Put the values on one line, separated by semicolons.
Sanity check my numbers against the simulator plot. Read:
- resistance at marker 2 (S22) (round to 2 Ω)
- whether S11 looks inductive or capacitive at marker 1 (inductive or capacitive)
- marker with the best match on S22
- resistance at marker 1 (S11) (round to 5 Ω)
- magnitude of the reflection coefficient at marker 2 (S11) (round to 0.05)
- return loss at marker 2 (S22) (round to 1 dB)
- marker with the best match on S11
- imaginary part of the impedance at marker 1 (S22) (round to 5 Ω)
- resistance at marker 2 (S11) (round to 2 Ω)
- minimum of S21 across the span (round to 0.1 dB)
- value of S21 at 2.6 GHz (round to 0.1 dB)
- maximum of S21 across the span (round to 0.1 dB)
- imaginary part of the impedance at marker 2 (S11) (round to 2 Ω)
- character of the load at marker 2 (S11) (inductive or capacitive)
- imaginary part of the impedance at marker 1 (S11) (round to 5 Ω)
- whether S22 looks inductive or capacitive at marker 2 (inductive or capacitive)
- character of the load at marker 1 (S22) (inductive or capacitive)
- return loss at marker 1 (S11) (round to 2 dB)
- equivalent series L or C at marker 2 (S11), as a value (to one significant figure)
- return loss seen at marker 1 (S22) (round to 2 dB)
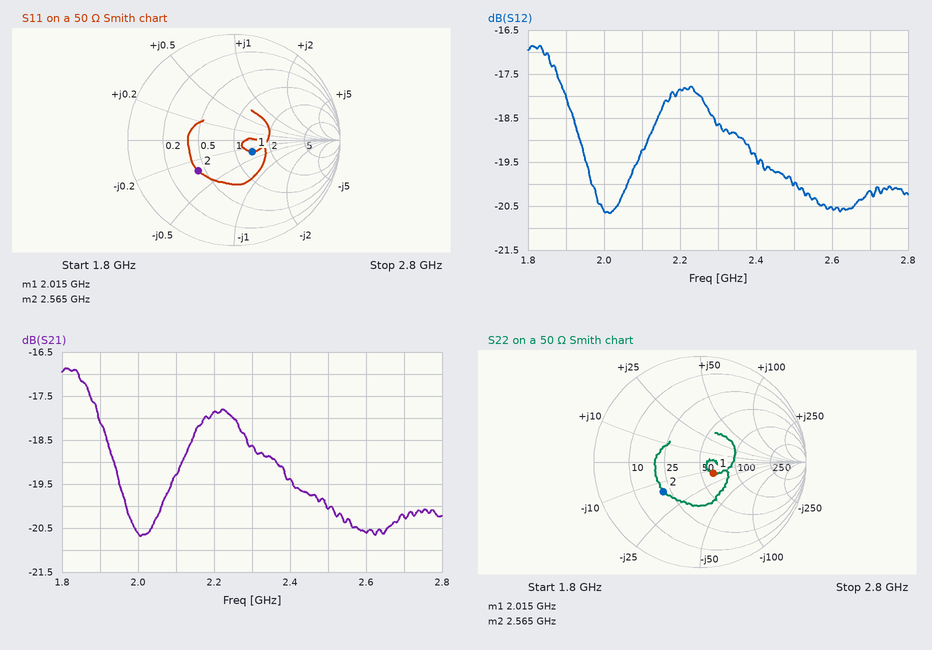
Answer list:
22 Ω; capacitive; marker 1; 70 Ω; 0.45; 7 dB; marker 1; -15 Ω; 22 Ω; -20.7 dB; -20.6 dB; -16.9 dB; -16 Ω; capacitive; -15 Ω; capacitive; capacitive; 14 dB; 4 pF; 16 dB
